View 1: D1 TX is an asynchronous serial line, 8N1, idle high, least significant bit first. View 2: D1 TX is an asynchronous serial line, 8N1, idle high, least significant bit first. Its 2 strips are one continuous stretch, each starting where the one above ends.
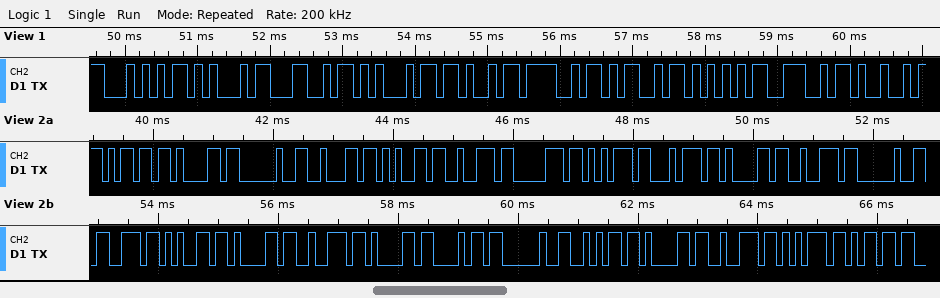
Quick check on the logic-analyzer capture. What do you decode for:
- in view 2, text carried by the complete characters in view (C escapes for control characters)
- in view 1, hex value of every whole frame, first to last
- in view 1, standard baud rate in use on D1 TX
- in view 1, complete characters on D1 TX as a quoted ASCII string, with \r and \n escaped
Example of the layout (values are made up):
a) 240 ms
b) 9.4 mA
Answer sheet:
a) "ma berputar searah jarum"
b) 54 45 4C 45 4B 4F 4D 55 4E 49
c) 9600 baud
d) "TELEKOMUNI"
